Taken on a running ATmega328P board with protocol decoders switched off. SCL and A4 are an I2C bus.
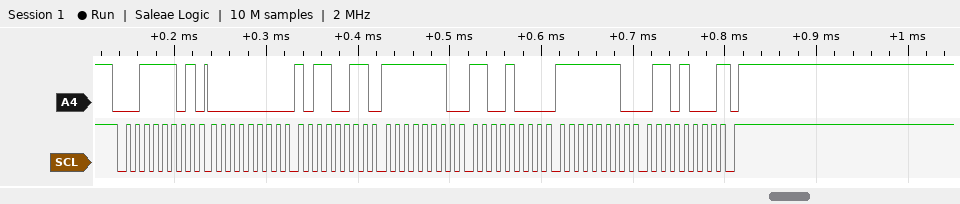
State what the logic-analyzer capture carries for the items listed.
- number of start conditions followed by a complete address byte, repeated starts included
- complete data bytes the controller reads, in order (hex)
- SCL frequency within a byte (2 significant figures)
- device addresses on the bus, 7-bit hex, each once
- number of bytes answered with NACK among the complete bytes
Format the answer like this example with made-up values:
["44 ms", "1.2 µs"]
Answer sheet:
["1", "00 B3 FE C8 FE 68", "100 kHz", "0x1E", "1"]
